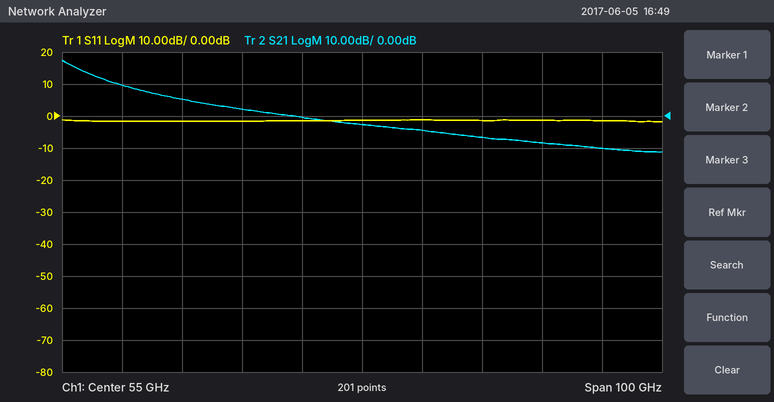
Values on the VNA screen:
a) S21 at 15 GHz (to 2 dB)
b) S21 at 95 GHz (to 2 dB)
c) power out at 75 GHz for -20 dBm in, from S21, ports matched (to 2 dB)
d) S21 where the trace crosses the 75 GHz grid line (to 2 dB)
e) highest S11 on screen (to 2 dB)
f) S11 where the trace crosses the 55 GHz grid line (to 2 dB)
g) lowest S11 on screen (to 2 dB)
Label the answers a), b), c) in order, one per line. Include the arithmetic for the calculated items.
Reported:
a) 10 dB
b) -10 dB
c) -20 dBm + (-6 dB) = -26 dBm
d) -6 dB
e) -2 dB
f) -2 dB
g) -2 dB
